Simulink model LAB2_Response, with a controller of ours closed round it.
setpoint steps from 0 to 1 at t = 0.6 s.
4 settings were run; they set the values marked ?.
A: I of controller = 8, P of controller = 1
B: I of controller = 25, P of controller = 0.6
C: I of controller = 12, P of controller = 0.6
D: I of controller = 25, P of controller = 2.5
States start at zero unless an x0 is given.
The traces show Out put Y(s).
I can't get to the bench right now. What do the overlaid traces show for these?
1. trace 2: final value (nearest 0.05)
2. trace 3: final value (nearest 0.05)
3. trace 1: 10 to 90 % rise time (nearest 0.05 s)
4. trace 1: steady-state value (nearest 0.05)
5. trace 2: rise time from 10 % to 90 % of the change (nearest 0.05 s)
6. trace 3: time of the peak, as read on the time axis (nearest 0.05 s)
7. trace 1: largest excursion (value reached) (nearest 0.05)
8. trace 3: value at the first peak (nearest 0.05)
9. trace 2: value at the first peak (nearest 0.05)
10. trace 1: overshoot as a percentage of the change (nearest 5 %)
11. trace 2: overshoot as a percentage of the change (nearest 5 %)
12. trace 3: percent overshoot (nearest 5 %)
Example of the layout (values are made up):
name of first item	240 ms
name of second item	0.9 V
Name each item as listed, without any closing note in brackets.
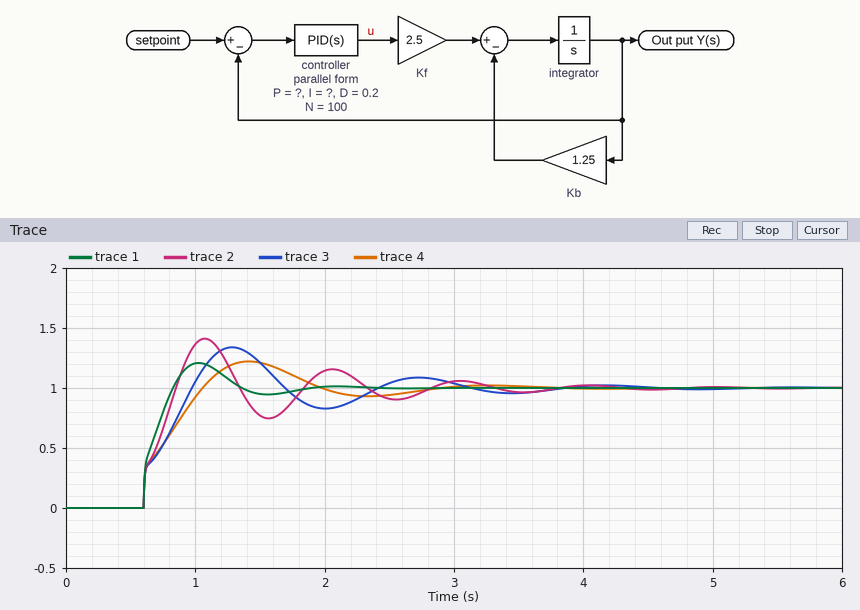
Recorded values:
trace 2: final value	1.00
trace 3: final value	1.00
trace 1: 10 to 90 % rise time	0.20 s
trace 1: steady-state value	1.00
trace 2: rise time from 10 % to 90 % of the change	0.20 s
trace 3: time of the peak, as read on the time axis	1.30 s
trace 1: largest excursion (value reached)	1.20
trace 3: value at the first peak	1.35
trace 2: value at the first peak	1.40
trace 1: overshoot as a percentage of the change	20 %
trace 2: overshoot as a percentage of the change	40 %
trace 3: percent overshoot	35 %
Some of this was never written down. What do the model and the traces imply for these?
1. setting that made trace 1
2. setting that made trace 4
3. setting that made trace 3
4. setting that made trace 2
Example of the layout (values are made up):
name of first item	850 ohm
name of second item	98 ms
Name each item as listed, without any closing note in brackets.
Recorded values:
setting that made trace 1	D
setting that made trace 4	A
setting that made trace 3	C
setting that made trace 2	B
